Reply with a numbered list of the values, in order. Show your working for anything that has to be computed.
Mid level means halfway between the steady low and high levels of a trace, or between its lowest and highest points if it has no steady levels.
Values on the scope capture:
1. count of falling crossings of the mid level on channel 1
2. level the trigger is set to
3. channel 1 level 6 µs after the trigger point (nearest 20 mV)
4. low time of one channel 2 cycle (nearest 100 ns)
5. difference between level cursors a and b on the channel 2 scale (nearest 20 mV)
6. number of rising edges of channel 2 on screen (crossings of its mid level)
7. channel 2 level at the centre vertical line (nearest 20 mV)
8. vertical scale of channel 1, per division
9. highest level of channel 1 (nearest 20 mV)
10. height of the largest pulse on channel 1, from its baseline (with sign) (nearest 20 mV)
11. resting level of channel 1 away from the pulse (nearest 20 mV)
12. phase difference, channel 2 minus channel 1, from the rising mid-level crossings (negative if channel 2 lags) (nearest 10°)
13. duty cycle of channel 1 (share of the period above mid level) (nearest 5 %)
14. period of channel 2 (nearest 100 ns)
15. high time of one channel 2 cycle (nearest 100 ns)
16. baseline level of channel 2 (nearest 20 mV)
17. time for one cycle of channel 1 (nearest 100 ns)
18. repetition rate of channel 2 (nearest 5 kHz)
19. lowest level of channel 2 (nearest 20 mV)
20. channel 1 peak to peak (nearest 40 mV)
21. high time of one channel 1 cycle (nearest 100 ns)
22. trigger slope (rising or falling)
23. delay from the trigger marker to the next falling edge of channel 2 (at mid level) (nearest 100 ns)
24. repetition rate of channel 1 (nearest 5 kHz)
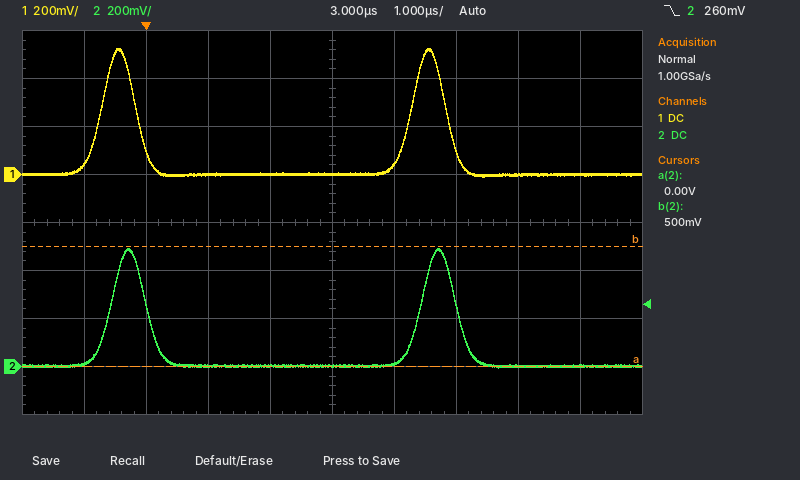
1. 2
2. 260 mV
3. 0 mV
4. 4.4 µs
5. 500 mV
6. 2
7. 0 mV
8. 200 mV
9. 520 mV
10. 520 mV − (0 mV) = +520 mV
11. 0 mV
12. -10°
13. 600 ns / 5.0 µs ≈ 12.0 %, so 10 % to the nearest 5 %
14. 5.0 µs
15. 600 ns
16. 0 mV
17. 5.0 µs
18. 1 / 5.0 µs ≈ 200 kHz
19. 0 mV
20. 520 mV
21. 600 ns
22. falling
23. 5.0 µs
24. 1 / 5.0 µs ≈ 200 kHz
